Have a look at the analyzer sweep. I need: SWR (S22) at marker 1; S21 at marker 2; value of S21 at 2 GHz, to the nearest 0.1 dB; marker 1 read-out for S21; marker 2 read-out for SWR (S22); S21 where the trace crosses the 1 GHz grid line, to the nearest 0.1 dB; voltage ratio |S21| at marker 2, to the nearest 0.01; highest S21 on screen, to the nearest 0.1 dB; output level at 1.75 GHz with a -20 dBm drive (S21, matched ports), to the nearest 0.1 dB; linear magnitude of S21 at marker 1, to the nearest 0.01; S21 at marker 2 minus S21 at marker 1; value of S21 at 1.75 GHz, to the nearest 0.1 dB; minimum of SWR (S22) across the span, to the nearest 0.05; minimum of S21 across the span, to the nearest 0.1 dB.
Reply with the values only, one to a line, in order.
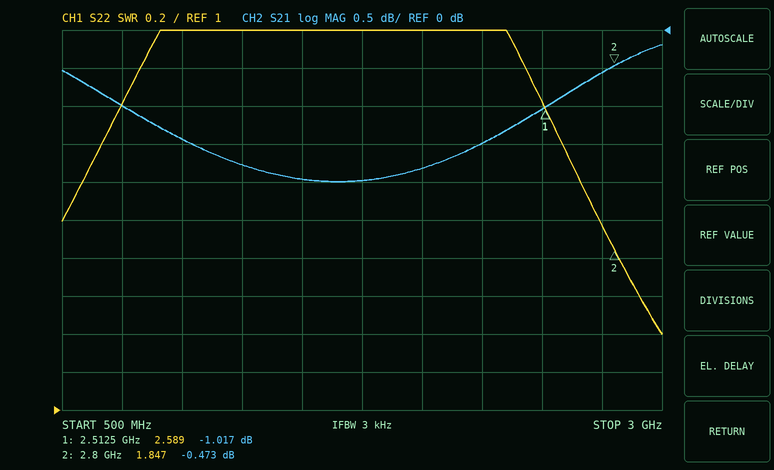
2.589
-0.473 dB
-1.8 dB
-1.017 dB
1.847
-1.4 dB
0.95
-0.2 dB
-22.0 dBm
0.89
0.544 dB
-2.0 dB
1.40
-2.0 dB
